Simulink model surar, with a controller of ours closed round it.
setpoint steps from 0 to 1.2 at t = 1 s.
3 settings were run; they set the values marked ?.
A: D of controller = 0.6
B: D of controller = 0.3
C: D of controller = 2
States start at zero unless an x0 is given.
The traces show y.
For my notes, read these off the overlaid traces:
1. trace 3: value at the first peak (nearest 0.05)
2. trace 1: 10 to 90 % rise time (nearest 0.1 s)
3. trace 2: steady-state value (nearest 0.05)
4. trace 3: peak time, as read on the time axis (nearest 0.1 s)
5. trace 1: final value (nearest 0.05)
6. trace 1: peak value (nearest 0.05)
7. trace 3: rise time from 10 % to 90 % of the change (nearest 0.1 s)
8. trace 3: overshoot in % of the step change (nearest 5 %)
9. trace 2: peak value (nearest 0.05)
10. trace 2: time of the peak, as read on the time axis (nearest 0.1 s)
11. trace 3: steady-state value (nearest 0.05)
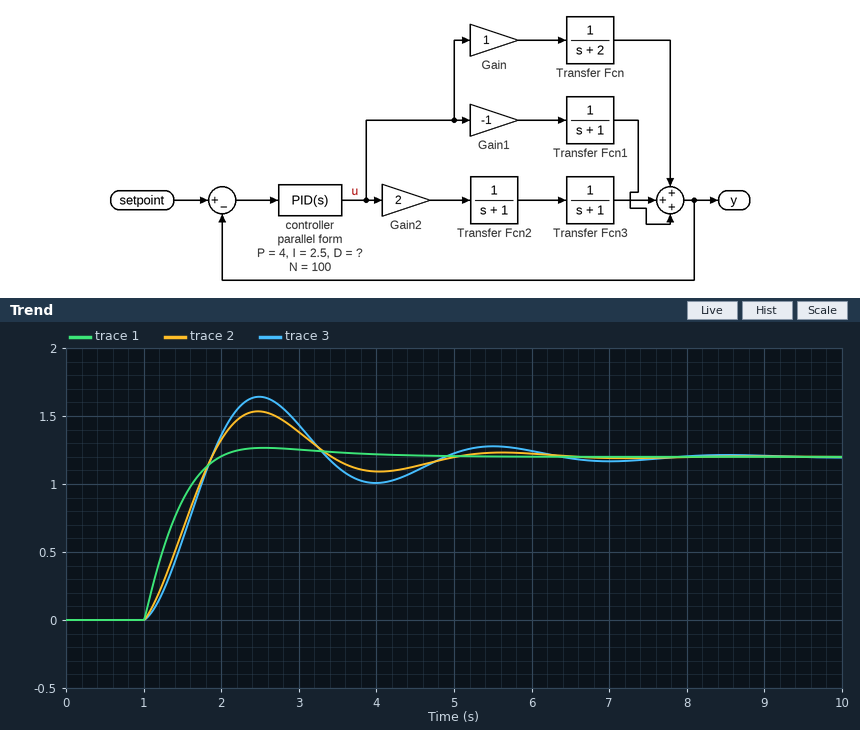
1.65
0.7 s
1.20
2.5 s
1.20
1.25
0.6 s
35 %
1.55
2.5 s
1.20
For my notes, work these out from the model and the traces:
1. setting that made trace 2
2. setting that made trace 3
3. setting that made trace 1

A
B
C
